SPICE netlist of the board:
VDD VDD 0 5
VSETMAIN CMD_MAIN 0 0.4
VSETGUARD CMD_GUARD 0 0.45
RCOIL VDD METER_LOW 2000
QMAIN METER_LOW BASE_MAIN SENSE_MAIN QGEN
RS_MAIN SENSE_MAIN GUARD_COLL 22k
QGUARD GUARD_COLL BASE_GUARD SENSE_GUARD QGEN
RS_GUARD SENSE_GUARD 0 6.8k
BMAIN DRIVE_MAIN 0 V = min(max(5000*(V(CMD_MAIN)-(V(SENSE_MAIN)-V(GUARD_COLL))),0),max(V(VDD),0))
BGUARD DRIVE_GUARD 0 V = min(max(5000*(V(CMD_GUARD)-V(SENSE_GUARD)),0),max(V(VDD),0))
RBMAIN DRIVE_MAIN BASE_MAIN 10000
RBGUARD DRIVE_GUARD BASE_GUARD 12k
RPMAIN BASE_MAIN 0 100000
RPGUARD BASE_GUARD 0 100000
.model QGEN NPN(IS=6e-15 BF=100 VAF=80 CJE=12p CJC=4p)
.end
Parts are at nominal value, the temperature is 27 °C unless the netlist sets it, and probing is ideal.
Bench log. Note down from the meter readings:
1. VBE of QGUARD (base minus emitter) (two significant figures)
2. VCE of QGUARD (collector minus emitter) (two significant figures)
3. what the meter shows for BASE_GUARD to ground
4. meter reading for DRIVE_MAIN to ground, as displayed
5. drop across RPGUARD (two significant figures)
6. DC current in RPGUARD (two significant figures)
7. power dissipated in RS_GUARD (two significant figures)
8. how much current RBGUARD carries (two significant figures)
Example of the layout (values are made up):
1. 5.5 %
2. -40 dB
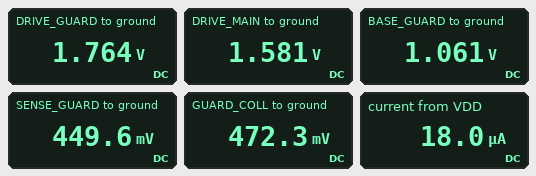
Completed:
1. 610 mV
2. 23 mV
3. 1.061 V
4. 1.581 V
5. 1.1 V
6. 11 µA
7. 30 µW
8. 59 µA
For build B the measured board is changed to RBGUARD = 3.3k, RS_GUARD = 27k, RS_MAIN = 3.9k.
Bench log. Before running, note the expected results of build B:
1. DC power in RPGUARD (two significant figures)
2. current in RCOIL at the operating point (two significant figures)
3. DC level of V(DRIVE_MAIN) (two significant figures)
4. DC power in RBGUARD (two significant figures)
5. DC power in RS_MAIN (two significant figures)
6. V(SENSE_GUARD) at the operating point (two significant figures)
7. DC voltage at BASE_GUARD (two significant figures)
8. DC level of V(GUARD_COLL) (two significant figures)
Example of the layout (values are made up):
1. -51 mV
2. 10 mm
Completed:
1. 10 µW
2. 16 µA
3. 5.0 V
4. 350 nW
5. 1.1 µW
6. 450 mV
7. 1.0 V
8. 3.9 V
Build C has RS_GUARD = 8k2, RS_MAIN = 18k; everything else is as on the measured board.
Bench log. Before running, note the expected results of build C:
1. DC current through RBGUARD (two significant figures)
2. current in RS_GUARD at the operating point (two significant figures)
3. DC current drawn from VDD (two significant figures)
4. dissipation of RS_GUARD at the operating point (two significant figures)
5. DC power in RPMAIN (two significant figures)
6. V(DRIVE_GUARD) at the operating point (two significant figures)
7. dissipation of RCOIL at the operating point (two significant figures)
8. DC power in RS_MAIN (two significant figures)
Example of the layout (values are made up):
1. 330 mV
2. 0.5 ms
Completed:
1. 43 µA
2. 55 µA
3. 22 µA
4. 25 µW
5. 21 µW
6. 1.6 V
7. 970 nW
8. 8.9 µW
